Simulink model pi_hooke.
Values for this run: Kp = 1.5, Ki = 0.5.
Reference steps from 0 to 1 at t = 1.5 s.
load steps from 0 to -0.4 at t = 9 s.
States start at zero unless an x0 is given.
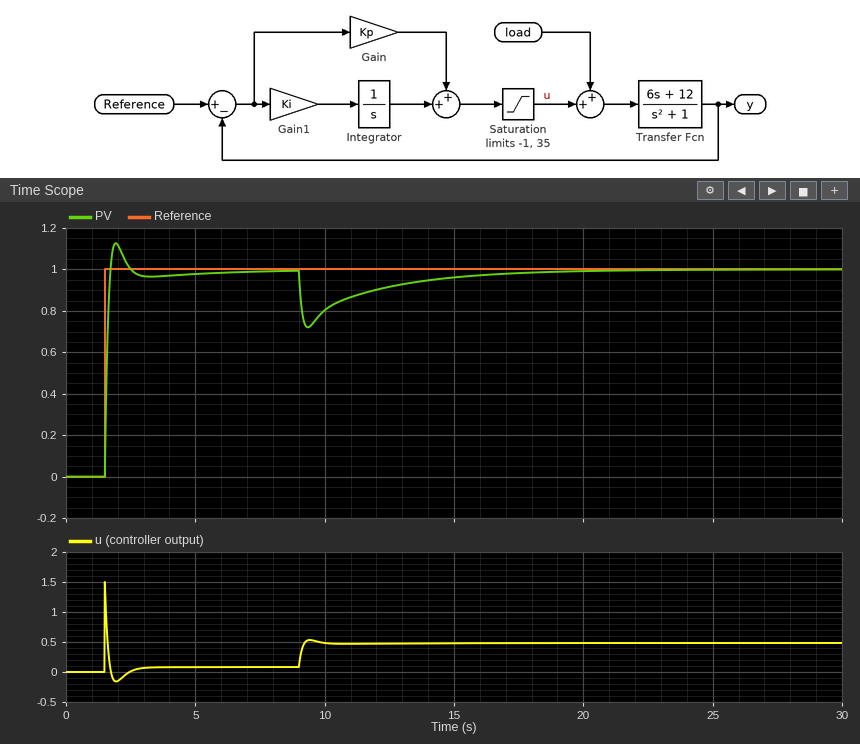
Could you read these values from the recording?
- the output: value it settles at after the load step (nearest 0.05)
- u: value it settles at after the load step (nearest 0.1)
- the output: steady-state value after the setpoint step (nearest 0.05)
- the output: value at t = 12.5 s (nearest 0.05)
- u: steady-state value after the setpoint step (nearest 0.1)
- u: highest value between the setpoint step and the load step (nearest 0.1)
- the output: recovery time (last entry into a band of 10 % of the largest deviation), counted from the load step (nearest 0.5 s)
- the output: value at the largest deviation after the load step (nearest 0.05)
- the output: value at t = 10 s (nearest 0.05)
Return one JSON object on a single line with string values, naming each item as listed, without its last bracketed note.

{"the output: value it settles at after the load step": "1.00", "u: value it settles at after the load step": "0.5", "the output: steady-state value after the setpoint step": "1.00", "the output: value at t = 12.5 s": "0.90", "u: steady-state value after the setpoint step": "0.1", "u: highest value between the setpoint step and the load step": "1.5", "the output: recovery time (last entry into a band of 10 % of the largest deviation), counted from the load step": "7.0 s", "the output: value at the largest deviation after the load step": "0.70", "the output: value at t = 10 s": "0.80"}
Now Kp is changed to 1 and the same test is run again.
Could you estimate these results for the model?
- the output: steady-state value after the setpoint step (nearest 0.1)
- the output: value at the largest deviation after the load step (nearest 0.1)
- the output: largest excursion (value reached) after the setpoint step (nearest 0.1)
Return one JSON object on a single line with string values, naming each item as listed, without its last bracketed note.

{"the output: steady-state value after the setpoint step": "1.0", "the output: value at the largest deviation after the load step": "0.6", "the output: largest excursion (value reached) after the setpoint step": "1.2"}
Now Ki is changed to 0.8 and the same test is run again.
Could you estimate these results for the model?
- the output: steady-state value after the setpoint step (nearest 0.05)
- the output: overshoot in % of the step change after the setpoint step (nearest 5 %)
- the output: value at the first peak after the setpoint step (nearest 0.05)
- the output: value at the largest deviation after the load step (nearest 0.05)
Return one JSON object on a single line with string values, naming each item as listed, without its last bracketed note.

{"the output: steady-state value after the setpoint step": "1.00", "the output: overshoot in % of the step change after the setpoint step": "15 %", "the output: value at the first peak after the setpoint step": "1.15", "the output: value at the largest deviation after the load step": "0.75"}
